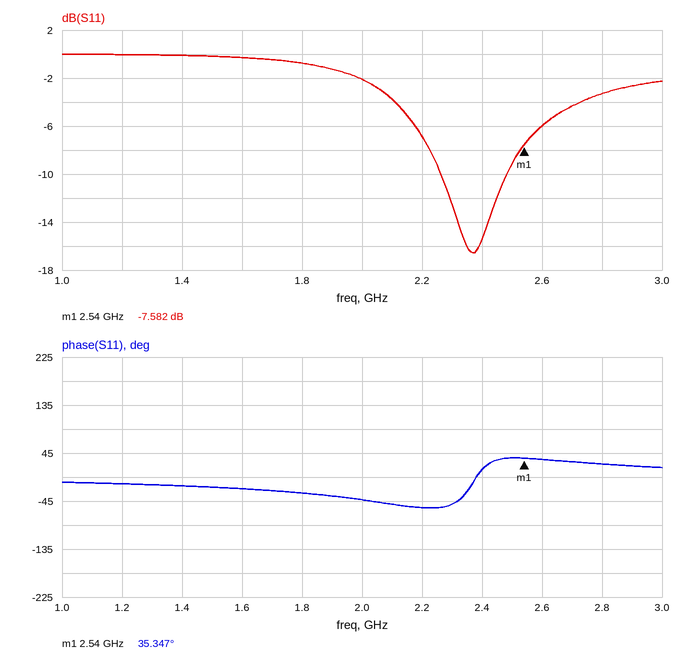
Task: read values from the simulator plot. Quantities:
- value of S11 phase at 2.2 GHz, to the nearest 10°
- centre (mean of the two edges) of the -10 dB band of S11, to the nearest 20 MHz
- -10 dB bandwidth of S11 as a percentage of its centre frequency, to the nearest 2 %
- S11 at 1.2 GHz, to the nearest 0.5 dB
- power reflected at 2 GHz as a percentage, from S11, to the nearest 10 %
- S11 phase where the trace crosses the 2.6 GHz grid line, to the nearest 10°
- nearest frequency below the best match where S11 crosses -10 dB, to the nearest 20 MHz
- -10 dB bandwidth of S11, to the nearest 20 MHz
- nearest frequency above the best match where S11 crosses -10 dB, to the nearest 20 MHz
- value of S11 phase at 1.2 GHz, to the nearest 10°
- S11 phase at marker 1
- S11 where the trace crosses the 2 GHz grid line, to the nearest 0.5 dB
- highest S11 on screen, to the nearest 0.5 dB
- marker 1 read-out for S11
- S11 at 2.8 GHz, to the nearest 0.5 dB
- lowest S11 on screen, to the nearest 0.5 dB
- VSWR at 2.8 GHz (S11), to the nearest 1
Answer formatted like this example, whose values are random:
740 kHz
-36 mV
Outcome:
-60°
2.38 GHz
10 %
0.0 dB
60 %
30°
2.26 GHz
220 MHz
2.48 GHz
-10°
35.347°
-2.0 dB
0.0 dB
-7.582 dB
-3.5 dB
-16.5 dB
5
